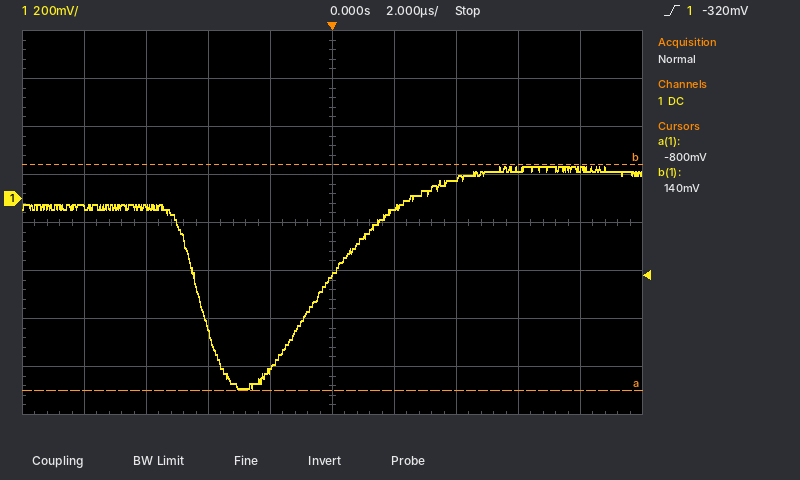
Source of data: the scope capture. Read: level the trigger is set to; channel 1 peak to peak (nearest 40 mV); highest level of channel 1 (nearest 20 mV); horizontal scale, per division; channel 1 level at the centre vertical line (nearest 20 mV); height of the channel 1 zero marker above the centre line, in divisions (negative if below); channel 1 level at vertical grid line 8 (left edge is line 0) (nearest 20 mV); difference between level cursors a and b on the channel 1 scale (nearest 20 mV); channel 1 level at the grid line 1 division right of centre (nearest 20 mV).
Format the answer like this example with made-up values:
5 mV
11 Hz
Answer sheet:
-320 mV
920 mV
140 mV
2 µs
-320 mV
+0.5 div
120 mV
940 mV
-40 mV
